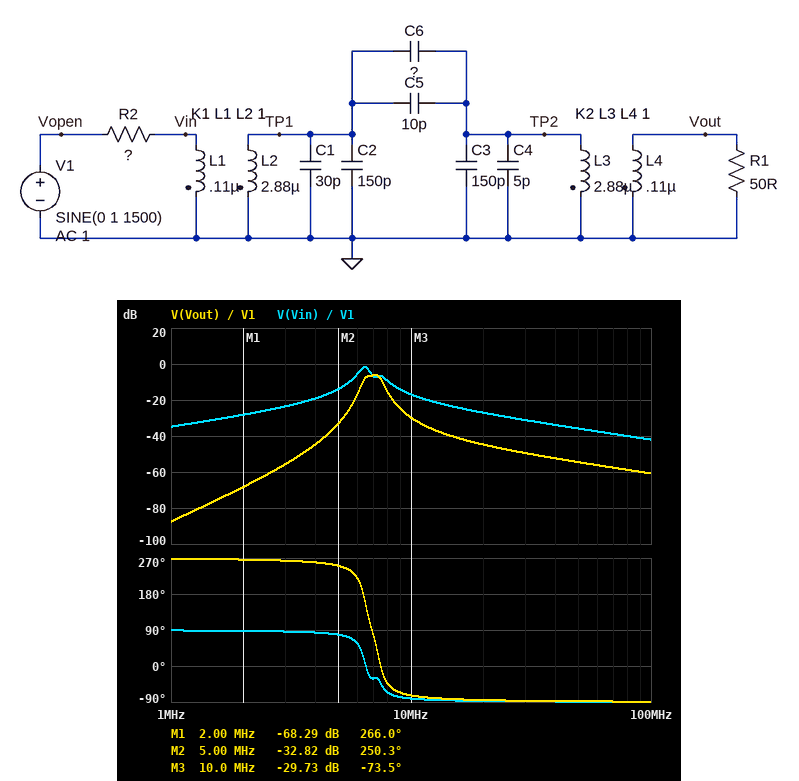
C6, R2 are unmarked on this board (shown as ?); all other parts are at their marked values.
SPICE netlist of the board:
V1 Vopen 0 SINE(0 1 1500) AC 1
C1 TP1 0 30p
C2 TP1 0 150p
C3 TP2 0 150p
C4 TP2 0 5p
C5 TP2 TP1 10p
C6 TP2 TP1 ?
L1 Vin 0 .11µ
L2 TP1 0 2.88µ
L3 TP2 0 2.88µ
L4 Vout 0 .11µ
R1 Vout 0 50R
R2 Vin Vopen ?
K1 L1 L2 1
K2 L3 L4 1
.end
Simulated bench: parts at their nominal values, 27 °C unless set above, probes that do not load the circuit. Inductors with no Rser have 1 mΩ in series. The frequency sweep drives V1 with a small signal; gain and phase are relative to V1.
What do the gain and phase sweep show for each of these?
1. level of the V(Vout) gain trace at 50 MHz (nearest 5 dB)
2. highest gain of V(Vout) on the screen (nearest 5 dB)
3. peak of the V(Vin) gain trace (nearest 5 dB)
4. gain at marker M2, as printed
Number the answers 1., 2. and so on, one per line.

1. -55 dB
2. -5 dB
3. 0 dB
4. -32.82 dB
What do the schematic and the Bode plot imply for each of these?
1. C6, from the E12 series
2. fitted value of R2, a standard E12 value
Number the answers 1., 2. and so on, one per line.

1. 10 pF
2. 39 Ω
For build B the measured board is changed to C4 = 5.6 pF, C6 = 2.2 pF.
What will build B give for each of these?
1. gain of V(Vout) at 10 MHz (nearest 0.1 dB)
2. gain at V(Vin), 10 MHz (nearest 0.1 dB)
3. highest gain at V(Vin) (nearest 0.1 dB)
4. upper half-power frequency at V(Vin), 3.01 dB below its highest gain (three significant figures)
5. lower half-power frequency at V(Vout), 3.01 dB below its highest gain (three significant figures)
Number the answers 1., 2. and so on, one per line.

1. -32.9 dB
2. -16.5 dB
3. -0.8 dB
4. 7.05 MHz
5. 6.61 MHz
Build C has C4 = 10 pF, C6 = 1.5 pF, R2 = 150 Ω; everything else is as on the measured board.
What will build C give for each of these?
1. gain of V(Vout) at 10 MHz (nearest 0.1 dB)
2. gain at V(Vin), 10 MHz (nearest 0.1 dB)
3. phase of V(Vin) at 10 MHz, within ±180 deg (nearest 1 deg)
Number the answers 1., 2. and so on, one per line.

1. -45.3 dB
2. -28.0 dB
3. -88 deg
